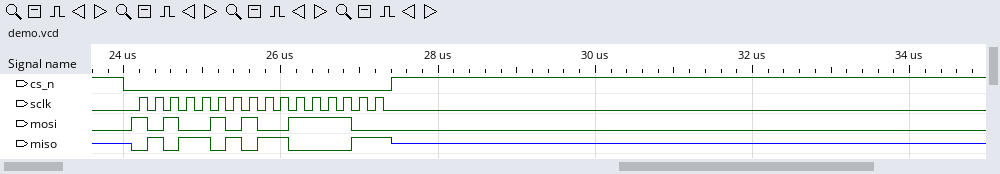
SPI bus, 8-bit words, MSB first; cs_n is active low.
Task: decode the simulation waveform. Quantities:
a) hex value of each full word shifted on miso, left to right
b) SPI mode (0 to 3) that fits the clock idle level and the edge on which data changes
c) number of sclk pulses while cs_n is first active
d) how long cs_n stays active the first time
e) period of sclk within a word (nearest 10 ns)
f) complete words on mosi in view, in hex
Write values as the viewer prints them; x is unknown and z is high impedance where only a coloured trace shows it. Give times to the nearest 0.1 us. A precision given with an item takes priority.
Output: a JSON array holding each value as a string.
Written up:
["5A, C3", "0", "16", "3.4 us", "200 ns", "A5, 3C"]
